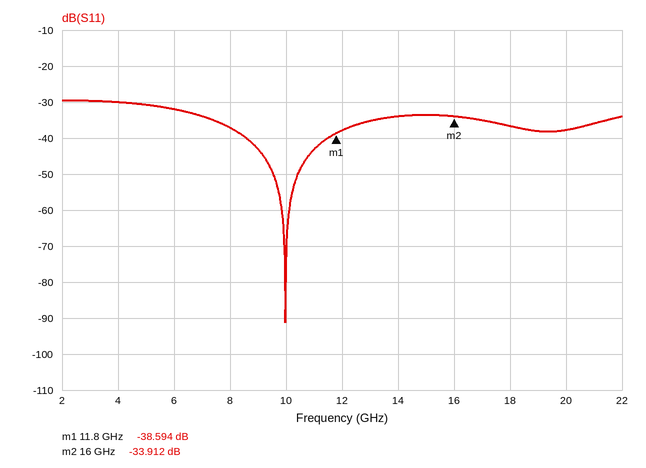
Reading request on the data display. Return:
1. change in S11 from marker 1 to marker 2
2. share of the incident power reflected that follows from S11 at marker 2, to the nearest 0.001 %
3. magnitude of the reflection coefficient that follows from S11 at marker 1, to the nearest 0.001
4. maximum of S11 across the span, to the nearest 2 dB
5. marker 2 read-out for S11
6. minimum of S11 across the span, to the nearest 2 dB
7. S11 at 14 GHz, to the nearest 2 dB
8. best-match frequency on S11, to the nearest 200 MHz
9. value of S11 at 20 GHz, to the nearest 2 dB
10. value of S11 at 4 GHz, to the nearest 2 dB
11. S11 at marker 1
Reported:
4.682 dB
0.041 %
0.012
-30 dB
-33.912 dB
-92 dB
-34 dB
10.0 GHz
-38 dB
-30 dB
-38.594 dB
